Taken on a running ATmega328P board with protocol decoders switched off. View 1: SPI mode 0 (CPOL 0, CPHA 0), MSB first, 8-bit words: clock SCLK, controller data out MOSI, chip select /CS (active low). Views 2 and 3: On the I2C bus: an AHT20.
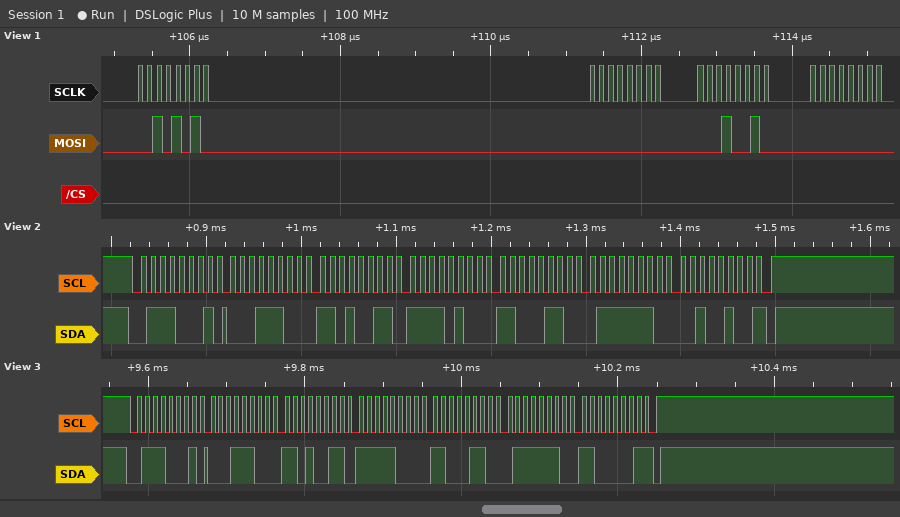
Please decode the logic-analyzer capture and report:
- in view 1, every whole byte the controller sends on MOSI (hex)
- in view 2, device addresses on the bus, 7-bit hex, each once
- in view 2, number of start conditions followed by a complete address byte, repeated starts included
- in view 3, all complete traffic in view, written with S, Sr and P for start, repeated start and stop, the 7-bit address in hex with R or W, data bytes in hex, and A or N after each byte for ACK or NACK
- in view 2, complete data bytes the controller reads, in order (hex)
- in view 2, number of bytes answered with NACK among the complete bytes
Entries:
2A 00 12 00
0x38
1
S 38R A 1C A D3 A F8 A C6 A 7E A C1 N P
1C D3 F4 C6 7E 24
1
